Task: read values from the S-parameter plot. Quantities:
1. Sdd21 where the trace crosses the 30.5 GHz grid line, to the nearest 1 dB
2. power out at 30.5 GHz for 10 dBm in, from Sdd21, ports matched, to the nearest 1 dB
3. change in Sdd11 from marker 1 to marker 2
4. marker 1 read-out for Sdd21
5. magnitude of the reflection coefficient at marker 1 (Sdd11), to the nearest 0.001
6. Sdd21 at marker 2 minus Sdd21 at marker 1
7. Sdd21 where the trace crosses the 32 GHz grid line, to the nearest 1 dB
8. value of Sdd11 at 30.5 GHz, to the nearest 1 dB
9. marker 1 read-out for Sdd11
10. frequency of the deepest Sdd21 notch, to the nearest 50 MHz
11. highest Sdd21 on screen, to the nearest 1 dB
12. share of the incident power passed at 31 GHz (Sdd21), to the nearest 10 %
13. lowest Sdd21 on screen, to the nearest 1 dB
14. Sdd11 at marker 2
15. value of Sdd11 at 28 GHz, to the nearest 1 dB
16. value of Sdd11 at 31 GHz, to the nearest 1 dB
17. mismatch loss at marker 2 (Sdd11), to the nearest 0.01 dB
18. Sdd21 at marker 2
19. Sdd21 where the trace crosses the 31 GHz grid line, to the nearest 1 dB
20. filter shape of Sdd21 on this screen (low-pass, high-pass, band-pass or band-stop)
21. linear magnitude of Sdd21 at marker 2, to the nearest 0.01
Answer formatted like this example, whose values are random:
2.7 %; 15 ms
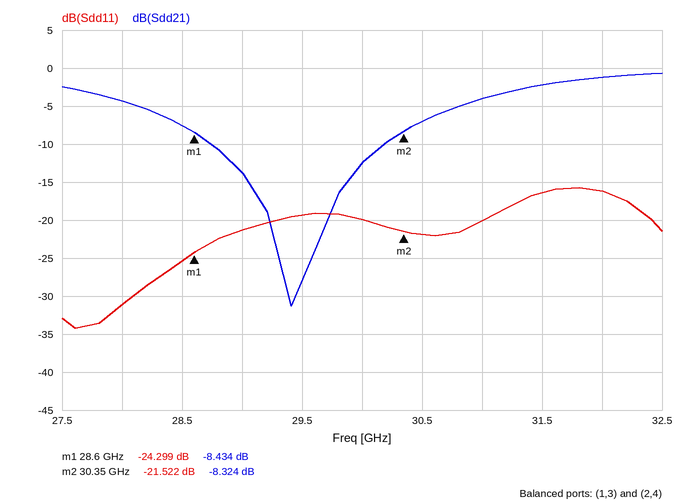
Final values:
-7 dB; 3 dBm; 2.777 dB; -8.434 dB; 0.061; 0.110 dB; -1 dB; -22 dB; -24.299 dB; 29.40 GHz; -1 dB; 40 %; -31 dB; -21.522 dB; -31 dB; -20 dB; 0.03 dB; -8.324 dB; -4 dB; band-stop; 0.38
